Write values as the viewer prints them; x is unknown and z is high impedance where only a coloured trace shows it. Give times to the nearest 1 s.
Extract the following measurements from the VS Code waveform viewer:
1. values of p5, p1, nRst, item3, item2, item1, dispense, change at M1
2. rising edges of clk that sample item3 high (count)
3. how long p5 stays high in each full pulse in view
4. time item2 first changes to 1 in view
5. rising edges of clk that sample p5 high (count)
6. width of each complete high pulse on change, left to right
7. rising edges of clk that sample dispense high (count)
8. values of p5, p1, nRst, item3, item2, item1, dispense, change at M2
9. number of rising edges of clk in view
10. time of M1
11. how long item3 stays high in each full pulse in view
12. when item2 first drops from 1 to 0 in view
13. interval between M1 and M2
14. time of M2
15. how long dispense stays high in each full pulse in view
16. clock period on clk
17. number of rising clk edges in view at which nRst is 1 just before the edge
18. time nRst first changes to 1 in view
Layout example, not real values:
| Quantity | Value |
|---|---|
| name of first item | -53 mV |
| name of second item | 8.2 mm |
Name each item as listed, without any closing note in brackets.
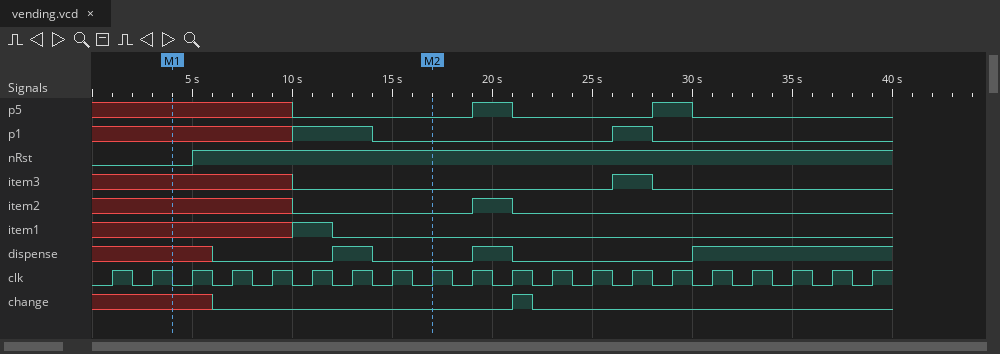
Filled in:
| Quantity | Value |
|---|---|
| values of p5, p1, nRst, item3, item2, item1, dispense, change at M1 | p5=x, p1=x, nRst=0, item3=x, item2=x, item1=x, dispense=x, change=x |
| rising edges of clk that sample item3 high | 1 |
| how long p5 stays high in each full pulse in view | 2 s, 2 s |
| time item2 first changes to 1 in view | 19 s |
| rising edges of clk that sample p5 high | 2 |
| width of each complete high pulse on change, left to right | 1 s |
| rising edges of clk that sample dispense high | 7 |
| values of p5, p1, nRst, item3, item2, item1, dispense, change at M2 | p5=0, p1=0, nRst=1, item3=0, item2=0, item1=0, dispense=0, change=0 |
| number of rising edges of clk in view | 20 |
| time of M1 | 4 s |
| how long item3 stays high in each full pulse in view | 2 s |
| when item2 first drops from 1 to 0 in view | 21 s |
| interval between M1 and M2 | 13 s |
| time of M2 | 17 s |
| how long dispense stays high in each full pulse in view | 2 s, 2 s |
| clock period on clk | 2 s |
| number of rising clk edges in view at which nRst is 1 just before the edge | 17 |
| time nRst first changes to 1 in view | 5 s |
